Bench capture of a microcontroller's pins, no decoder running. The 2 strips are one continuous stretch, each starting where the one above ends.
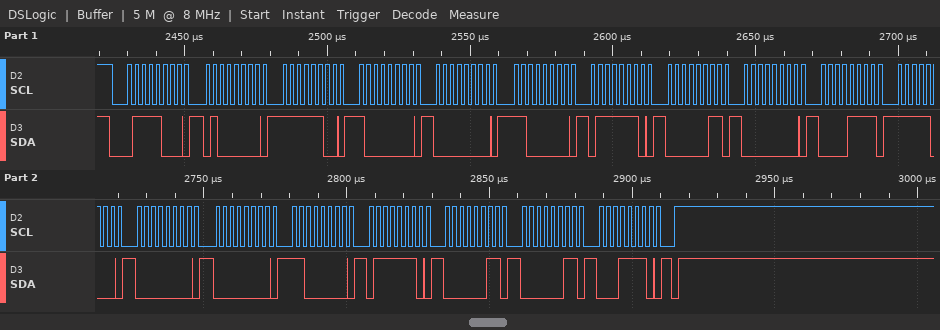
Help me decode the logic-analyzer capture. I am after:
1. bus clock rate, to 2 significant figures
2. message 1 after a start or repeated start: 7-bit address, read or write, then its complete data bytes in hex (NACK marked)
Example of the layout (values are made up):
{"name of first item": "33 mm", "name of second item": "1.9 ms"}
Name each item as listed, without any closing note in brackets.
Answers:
{"bus clock rate, to 2 significant figures": "400 kHz", "message 1 after a start or repeated start: 7-bit address, read or write, then its complete data bytes in hex": "0x3C write: 40 FC 80 00 C0 7E 03 00 0F F8 00 00 C0 7E 03 03 1E"}
